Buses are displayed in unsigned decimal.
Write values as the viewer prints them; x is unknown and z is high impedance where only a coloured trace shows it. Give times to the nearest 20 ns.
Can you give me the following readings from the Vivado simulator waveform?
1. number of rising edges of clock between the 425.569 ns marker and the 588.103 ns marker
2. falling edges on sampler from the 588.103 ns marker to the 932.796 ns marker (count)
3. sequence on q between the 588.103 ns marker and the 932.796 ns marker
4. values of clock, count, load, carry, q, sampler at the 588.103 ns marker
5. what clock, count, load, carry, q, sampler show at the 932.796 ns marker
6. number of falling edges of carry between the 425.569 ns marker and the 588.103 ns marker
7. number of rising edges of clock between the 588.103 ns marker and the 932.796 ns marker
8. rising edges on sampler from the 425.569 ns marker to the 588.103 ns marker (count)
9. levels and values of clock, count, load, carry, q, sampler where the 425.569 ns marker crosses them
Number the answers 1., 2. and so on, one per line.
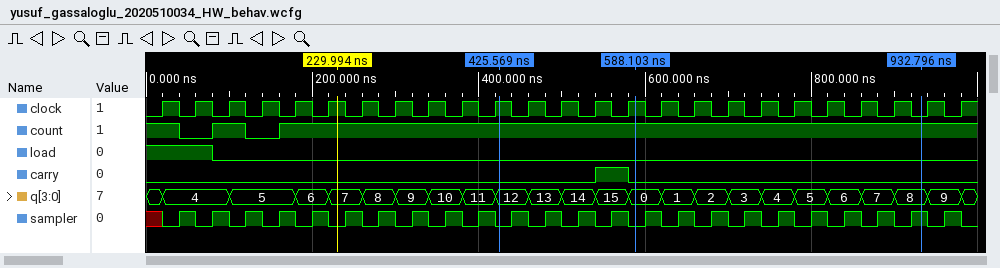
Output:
1. 4
2. 8
3. 0, 1, 2, 3, 4, 5, 6, 7, 8
4. clock=1, count=1, load=0, carry=0, q=0, sampler=0
5. clock=0, count=1, load=0, carry=0, q=8, sampler=1
6. 1
7. 8
8. 4
9. clock=1, count=1, load=0, carry=0, q=12, sampler=0
